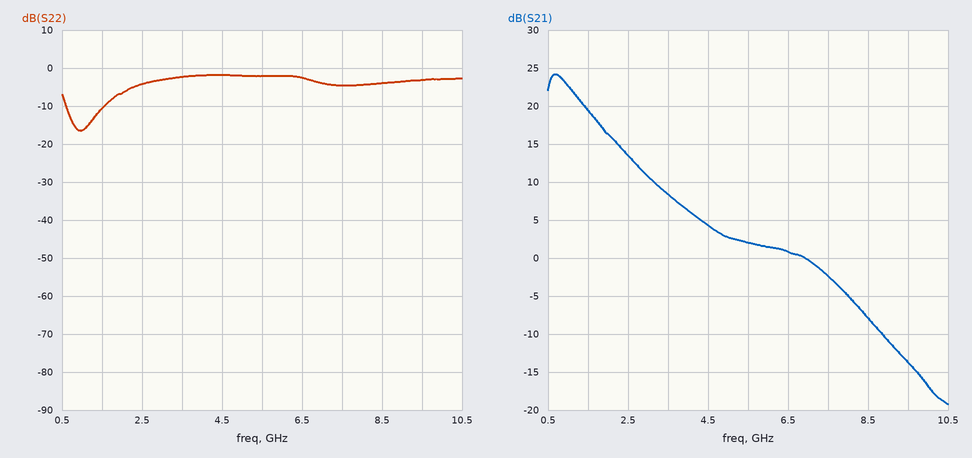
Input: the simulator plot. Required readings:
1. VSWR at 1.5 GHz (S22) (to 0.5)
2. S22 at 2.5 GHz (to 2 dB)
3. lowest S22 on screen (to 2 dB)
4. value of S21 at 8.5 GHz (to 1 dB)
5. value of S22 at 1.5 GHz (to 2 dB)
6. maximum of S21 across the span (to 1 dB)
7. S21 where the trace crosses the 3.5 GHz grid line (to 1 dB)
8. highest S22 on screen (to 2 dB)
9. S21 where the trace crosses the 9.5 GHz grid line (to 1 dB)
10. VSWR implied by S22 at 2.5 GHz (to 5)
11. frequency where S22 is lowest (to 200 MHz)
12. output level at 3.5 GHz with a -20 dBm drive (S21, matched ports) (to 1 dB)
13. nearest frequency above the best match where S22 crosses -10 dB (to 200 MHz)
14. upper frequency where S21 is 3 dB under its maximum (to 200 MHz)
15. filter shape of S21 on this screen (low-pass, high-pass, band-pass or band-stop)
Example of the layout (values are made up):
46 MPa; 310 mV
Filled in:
2.0; -4 dB; -16 dB; -8 dB; -10 dB; 24 dB; 8 dB; -2 dB; -14 dB; 5; 1.0 GHz; -12 dBm; 1.6 GHz; 1.2 GHz; low-pass
